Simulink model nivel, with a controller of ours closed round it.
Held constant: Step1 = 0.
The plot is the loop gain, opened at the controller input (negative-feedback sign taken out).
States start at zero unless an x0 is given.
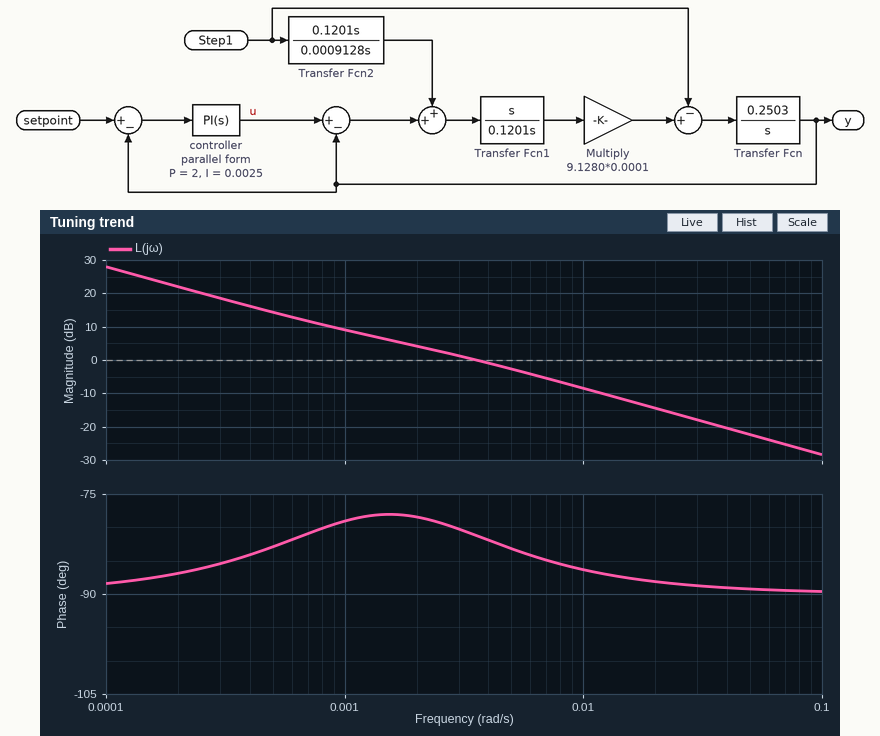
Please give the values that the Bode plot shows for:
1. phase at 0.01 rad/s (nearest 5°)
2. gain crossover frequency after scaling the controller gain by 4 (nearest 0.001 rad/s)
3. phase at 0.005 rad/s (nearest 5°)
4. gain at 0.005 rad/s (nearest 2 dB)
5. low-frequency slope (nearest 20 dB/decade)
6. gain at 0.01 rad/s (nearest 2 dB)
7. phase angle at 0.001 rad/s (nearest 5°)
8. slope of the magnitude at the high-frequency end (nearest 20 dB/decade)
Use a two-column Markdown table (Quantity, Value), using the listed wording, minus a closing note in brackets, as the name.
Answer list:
| Quantity | Value |
|---|---|
| phase at 0.01 rad/s | -85° |
| gain crossover frequency after scaling the controller gain by 4 | 0.015 rad/s |
| phase at 0.005 rad/s | -85° |
| gain at 0.005 rad/s | -2 dB |
| low-frequency slope | -20 dB/decade |
| gain at 0.01 rad/s | -8 dB |
| phase angle at 0.001 rad/s | -80° |
| slope of the magnitude at the high-frequency end | -20 dB/decade |
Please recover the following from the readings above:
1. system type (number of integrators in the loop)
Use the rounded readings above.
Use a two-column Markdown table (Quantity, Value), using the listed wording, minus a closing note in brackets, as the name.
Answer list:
| Quantity | Value |
|---|---|
| system type | 1 |
